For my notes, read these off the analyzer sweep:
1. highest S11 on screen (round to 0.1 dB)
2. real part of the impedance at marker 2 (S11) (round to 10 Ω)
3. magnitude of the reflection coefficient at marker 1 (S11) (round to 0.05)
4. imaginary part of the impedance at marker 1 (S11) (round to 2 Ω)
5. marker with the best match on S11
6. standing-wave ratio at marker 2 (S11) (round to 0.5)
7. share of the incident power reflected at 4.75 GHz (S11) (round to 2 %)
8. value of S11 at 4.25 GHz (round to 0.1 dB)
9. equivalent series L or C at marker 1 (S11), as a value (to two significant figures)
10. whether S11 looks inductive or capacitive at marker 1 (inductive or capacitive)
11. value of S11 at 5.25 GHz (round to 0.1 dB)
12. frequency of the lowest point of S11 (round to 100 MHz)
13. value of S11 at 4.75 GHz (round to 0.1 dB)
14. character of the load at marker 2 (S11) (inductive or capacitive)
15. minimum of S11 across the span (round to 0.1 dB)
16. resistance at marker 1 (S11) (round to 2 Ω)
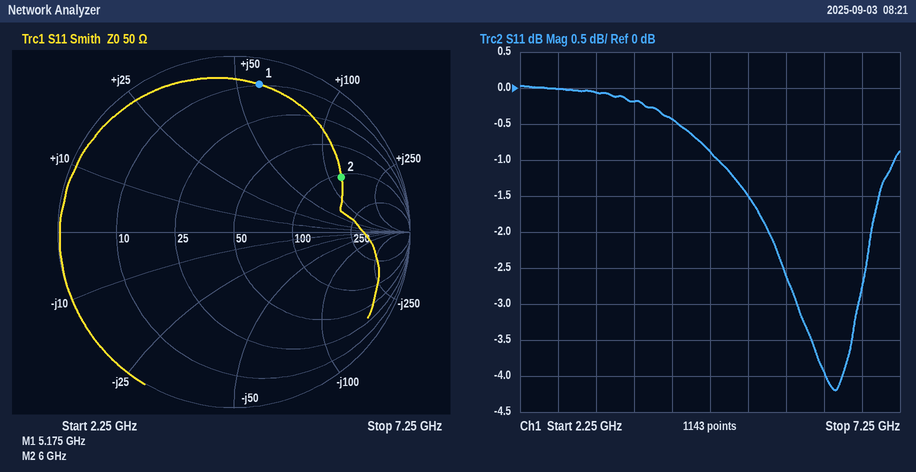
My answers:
0.0 dB
110 Ω
0.85
+58 Ω
marker 2
5.5
82 %
-0.4 dB
1.8 nH
inductive
-1.5 dB
6.4 GHz
-0.9 dB
inductive
-4.2 dB
10 Ω
